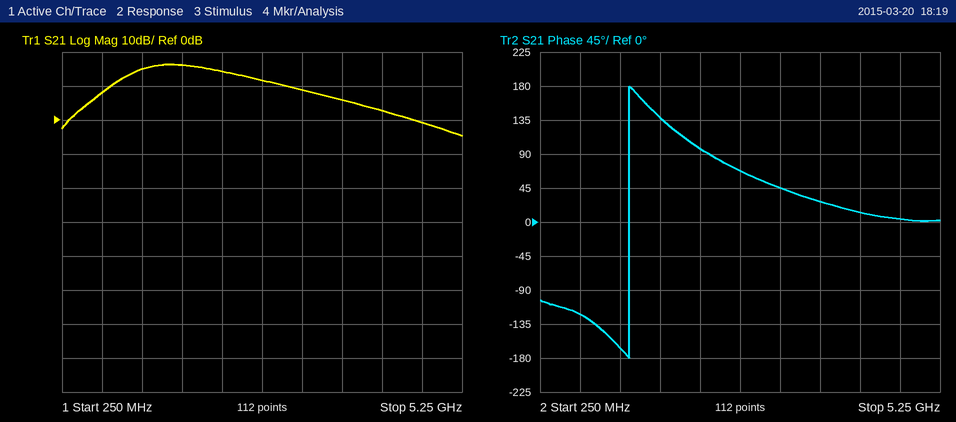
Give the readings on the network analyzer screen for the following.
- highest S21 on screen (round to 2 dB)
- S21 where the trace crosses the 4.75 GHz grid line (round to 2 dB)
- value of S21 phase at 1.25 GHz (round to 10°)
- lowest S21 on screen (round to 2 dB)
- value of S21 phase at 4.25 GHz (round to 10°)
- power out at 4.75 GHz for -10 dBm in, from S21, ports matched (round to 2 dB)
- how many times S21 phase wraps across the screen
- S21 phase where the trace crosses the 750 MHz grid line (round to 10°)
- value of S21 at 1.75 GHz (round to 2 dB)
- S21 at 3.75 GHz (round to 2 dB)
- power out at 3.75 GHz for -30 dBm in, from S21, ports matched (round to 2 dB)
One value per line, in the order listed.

16 dB
0 dB
-170°
-4 dB
10°
-10 dBm
1
-120°
16 dB
6 dB
-24 dBm
